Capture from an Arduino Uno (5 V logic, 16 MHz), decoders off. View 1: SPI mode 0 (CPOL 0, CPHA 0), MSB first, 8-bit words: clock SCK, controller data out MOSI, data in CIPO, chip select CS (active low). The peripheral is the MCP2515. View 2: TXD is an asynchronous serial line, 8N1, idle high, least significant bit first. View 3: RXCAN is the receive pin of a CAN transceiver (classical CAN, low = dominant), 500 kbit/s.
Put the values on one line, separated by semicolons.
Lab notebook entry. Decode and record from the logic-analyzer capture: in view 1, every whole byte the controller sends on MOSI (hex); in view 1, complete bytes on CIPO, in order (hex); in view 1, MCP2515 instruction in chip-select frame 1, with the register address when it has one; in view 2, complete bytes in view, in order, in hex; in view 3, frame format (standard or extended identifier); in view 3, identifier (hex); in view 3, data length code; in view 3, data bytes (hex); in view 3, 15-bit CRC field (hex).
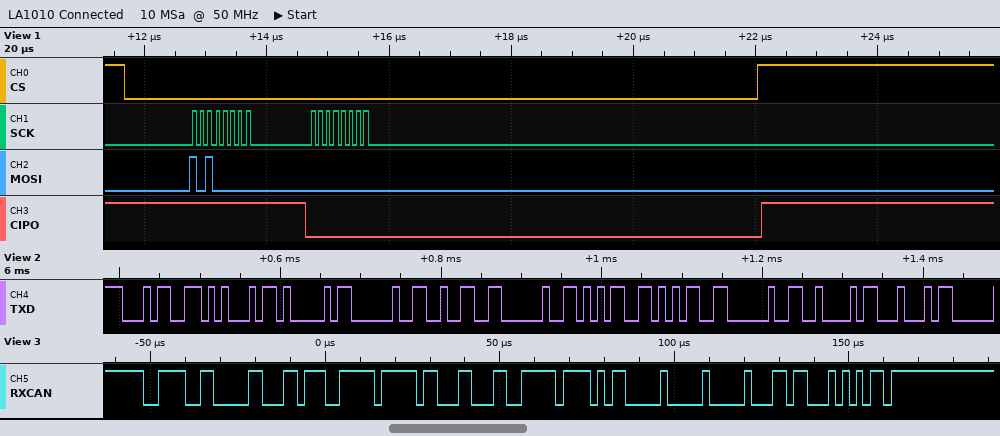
0xA0 0x00; 0xFF 0x00; READ STATUS; 0x34 0x45 0x41 0x20 0x32 0x20 0x35 0x35 0x20 0x42 0x44; standard; 0x3CC; 8; DC FF F1 8C FF AC 00 00; 0x6C55
